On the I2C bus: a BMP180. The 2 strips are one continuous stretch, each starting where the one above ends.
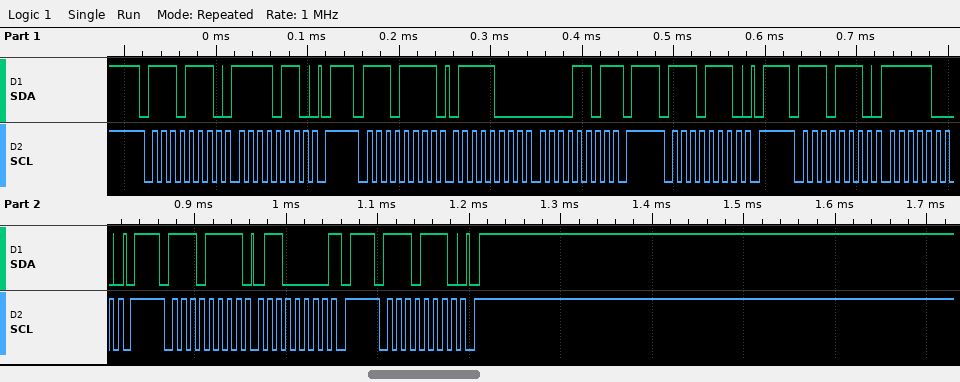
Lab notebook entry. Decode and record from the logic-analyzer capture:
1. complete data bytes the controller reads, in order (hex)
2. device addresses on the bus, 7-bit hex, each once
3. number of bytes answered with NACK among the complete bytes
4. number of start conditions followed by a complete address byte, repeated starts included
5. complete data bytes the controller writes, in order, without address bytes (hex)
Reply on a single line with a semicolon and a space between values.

78 0D 60; 0x77; 2; 6; F6 F8
